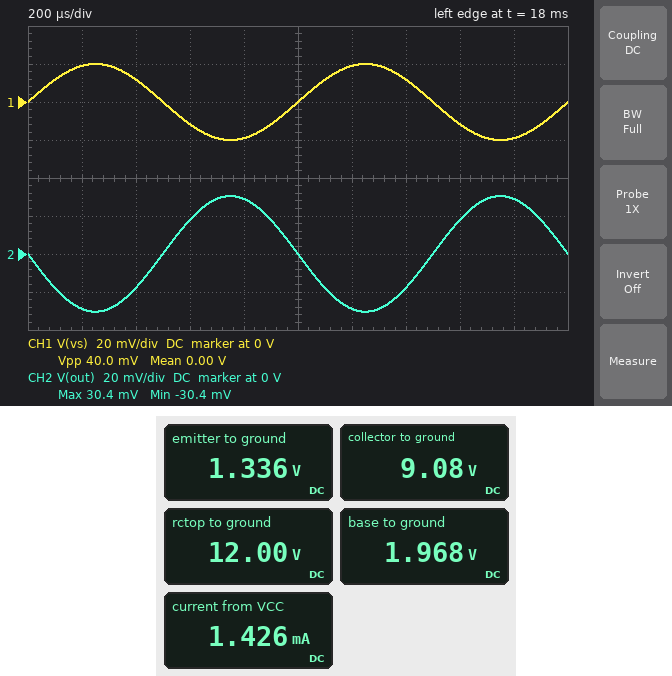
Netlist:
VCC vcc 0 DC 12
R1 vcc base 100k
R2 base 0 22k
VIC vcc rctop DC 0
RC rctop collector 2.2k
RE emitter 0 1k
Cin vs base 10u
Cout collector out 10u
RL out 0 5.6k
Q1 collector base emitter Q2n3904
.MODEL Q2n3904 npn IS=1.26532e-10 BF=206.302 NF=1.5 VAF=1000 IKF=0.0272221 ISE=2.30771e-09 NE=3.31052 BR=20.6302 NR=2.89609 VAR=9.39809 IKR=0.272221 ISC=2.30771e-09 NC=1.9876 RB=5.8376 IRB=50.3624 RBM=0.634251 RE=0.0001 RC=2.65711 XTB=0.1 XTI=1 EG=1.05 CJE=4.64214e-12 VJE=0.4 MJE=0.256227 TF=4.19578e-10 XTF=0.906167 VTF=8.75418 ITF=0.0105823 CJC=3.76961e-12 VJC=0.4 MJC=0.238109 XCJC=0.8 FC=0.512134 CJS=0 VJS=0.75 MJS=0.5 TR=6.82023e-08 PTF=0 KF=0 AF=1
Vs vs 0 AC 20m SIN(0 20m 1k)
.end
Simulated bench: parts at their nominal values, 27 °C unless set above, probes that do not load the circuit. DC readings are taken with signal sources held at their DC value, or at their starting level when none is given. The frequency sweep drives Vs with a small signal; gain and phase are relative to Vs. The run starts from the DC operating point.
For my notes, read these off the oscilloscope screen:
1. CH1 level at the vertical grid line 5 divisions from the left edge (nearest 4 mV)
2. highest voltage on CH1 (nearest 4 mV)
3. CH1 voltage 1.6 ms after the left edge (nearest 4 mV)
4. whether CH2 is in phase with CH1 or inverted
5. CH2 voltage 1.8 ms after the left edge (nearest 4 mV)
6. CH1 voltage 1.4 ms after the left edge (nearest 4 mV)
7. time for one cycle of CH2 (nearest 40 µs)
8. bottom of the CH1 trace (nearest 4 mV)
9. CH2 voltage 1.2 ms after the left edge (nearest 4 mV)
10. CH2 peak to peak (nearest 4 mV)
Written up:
0 V
20 mV
-12 mV
inverted
28 mV
12 mV
1.00 ms
-20 mV
-28 mV
60 mV
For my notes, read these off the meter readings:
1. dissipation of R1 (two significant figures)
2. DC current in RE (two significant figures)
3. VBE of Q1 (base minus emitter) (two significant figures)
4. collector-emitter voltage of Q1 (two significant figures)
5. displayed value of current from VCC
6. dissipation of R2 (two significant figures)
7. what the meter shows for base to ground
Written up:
1.0 mW
1.3 mA
630 mV
7.7 V
1.426 mA
180 µW
1.968 V
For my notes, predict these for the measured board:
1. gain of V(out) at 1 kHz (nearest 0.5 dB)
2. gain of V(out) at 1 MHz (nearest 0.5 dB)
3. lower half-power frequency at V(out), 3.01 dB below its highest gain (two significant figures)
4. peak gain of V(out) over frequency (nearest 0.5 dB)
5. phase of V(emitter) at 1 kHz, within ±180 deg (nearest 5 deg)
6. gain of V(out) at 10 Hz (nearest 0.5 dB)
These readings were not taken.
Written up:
3.5 dB
3.5 dB
2.4 Hz
3.5 dB
0 deg
3.5 dB
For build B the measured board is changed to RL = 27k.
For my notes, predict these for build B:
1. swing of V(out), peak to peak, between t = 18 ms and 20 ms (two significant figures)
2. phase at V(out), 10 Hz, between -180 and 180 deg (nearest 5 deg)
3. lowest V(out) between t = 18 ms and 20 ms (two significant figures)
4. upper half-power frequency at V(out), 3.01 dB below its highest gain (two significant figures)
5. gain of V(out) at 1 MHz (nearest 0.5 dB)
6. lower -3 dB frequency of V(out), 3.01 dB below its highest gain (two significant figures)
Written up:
78 mV
-170 deg
-39 mV
86 MHz
6.0 dB
1.2 Hz
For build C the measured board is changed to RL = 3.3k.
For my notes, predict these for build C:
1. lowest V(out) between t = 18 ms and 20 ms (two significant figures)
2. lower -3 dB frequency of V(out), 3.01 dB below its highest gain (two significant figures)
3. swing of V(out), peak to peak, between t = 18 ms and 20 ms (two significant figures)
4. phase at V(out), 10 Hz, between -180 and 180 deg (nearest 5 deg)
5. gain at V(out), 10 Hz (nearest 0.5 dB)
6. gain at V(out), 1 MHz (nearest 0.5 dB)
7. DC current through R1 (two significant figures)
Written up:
-25 mV
3.2 Hz
51 mV
-160 deg
1.5 dB
2.0 dB
100 µA
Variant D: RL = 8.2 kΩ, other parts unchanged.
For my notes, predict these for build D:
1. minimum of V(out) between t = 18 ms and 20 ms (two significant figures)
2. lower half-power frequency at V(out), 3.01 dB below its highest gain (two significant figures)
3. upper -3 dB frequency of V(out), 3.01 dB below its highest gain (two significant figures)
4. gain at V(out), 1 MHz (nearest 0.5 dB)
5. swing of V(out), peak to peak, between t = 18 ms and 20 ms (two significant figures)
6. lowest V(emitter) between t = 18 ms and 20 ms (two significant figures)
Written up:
-33 mV
2.0 Hz
200 MHz
4.5 dB
67 mV
1.3 V
